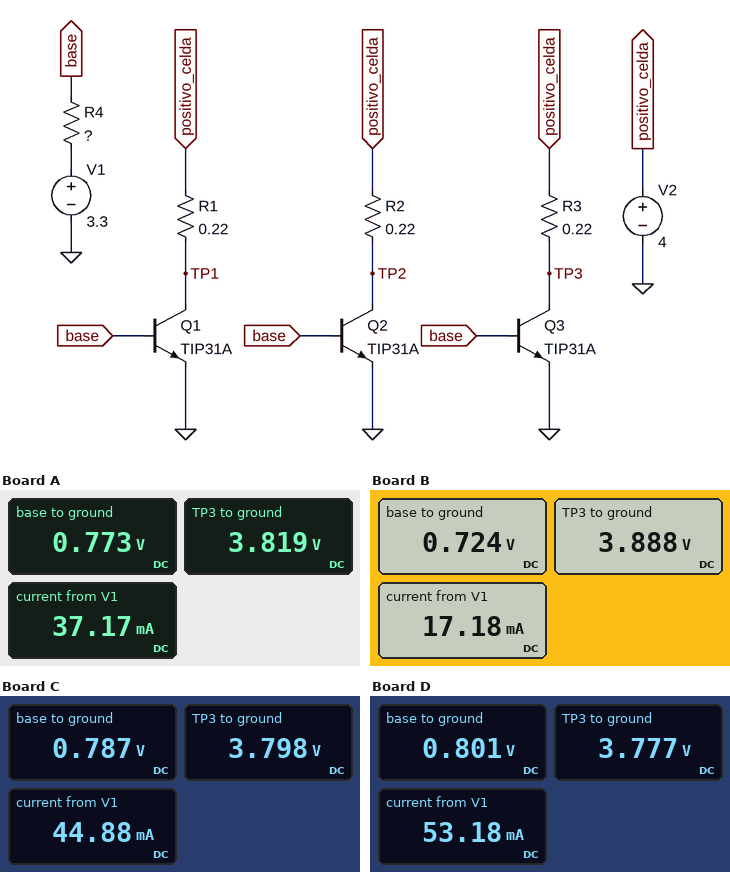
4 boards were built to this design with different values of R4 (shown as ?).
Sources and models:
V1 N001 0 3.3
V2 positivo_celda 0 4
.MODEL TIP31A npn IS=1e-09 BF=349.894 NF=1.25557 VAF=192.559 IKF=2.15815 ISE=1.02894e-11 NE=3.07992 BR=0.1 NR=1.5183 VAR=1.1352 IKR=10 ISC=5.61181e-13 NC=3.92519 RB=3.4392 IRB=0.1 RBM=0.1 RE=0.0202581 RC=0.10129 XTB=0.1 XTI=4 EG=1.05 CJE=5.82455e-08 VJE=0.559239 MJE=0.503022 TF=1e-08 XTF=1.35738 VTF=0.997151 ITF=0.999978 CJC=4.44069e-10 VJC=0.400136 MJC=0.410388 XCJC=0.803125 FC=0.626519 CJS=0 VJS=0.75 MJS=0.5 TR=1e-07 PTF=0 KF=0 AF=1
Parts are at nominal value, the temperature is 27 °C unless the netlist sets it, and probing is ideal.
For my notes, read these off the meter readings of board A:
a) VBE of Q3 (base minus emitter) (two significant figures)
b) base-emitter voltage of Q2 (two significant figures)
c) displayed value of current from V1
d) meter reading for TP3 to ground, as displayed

770 mV
770 mV
37.17 mA
3.819 V
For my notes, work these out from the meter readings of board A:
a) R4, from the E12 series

68 Ω
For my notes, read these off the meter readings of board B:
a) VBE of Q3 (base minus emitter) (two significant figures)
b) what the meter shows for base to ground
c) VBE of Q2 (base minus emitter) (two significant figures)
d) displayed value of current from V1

720 mV
0.724 V
720 mV
17.18 mA
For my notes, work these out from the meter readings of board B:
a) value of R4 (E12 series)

150 Ω
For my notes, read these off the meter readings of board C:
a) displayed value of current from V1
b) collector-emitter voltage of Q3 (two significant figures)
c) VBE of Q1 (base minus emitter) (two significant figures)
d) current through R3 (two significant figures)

44.88 mA
3.8 V
790 mV
920 mA
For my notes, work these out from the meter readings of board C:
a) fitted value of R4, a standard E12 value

56 Ω
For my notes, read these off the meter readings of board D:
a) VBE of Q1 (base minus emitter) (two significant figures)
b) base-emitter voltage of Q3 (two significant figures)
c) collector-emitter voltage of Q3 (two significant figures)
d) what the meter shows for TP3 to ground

800 mV
800 mV
3.8 V
3.777 V
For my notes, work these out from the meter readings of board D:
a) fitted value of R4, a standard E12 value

47 Ω
